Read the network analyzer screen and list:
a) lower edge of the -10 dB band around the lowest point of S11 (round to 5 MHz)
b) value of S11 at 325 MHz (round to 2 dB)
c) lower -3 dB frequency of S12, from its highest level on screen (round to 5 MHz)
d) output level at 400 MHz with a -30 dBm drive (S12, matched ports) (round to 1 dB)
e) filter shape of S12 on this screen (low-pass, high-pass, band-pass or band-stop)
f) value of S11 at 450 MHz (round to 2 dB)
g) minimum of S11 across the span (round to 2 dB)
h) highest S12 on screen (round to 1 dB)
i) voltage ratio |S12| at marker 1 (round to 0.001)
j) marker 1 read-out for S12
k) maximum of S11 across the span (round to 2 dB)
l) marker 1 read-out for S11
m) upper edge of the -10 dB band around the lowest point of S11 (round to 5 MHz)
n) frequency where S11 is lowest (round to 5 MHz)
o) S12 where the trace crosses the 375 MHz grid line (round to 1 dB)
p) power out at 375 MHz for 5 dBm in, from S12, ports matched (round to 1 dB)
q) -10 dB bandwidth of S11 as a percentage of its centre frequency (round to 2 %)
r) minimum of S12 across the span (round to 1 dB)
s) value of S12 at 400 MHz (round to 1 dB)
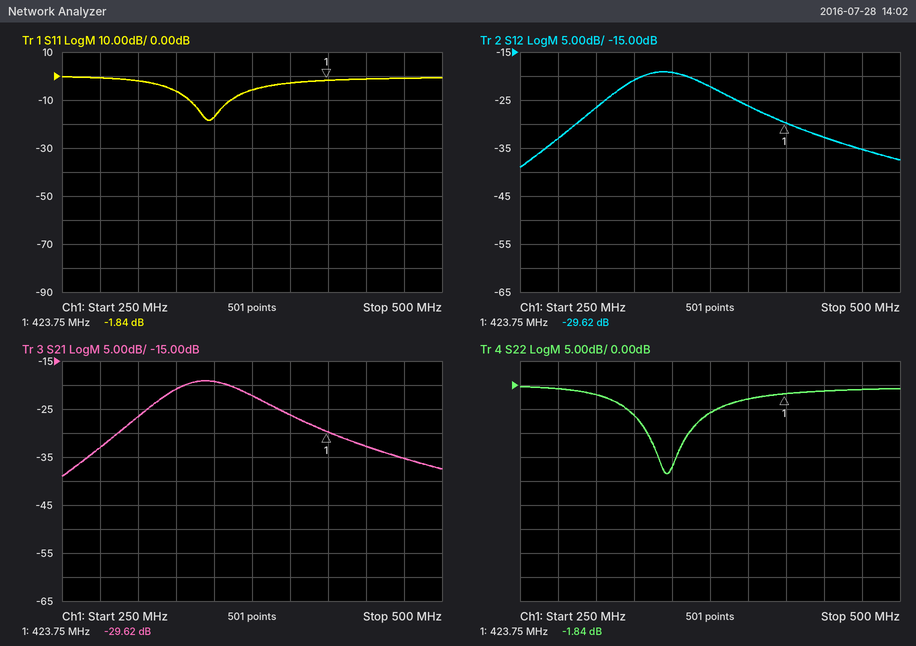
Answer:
335 MHz
-6 dB
320 MHz
-56 dBm
band-pass
-2 dB
-18 dB
-19 dB
0.033
-29.62 dB
0 dB
-1.84 dB
360 MHz
345 MHz
-22 dB
-17 dBm
8 %
-39 dB
-26 dB
